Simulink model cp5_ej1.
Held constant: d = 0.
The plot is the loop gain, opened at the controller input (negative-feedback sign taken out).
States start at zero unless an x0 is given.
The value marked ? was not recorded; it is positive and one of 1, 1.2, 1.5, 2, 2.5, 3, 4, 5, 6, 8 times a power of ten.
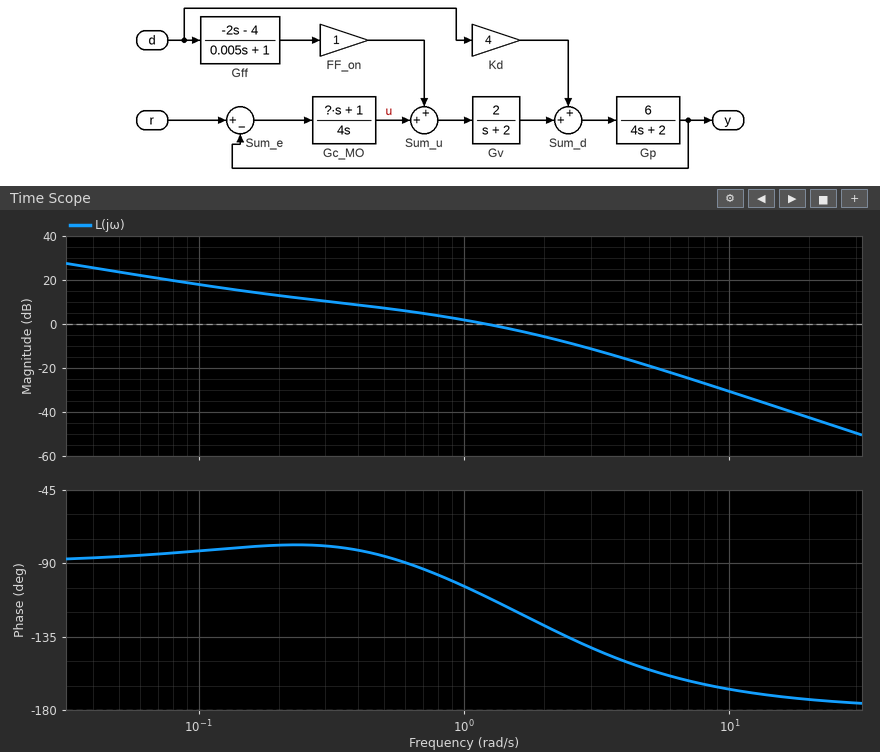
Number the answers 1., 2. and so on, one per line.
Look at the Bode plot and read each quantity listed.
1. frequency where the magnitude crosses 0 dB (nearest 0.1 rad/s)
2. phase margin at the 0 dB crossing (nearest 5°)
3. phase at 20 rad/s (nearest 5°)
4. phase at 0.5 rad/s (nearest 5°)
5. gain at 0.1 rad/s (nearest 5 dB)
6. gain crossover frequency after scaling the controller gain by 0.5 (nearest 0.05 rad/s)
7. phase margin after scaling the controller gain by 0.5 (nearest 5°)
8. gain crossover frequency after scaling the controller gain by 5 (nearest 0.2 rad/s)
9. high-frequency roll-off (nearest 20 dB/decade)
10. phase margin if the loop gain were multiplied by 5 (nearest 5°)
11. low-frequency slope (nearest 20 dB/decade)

1. 1.2 rad/s
2. 70°
3. -175°
4. -85°
5. 20 dB
6. 0.60 rad/s
7. 90°
8. 3.6 rad/s
9. -40 dB/decade
10. 35°
11. -20 dB/decade
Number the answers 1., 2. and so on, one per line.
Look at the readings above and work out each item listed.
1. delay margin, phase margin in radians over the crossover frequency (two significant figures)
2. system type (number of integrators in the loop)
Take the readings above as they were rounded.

1. 1.0 s
2. 1
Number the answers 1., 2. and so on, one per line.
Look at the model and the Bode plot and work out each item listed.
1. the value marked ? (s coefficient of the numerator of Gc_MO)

1. 4
